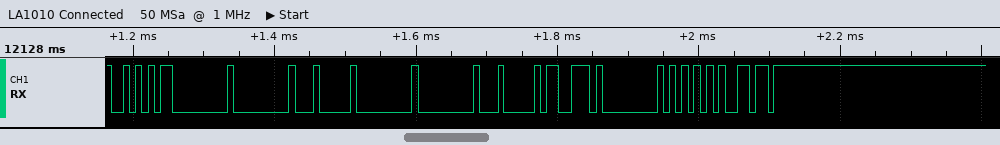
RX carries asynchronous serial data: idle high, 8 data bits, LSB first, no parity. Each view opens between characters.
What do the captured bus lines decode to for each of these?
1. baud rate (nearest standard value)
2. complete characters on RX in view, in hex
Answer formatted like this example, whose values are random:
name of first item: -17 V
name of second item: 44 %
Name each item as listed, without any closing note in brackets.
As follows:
baud rate: 115200 baud
complete characters on RX in view, in hex: AA, 00, 00, 04, 00, 00, 04, 73, 00, 55, B6
